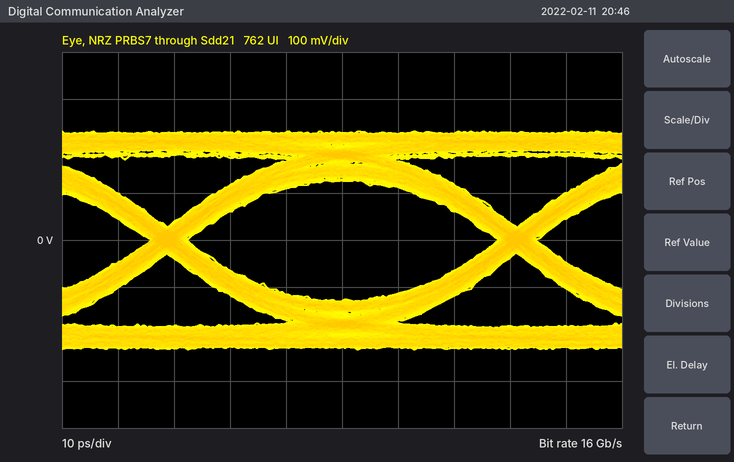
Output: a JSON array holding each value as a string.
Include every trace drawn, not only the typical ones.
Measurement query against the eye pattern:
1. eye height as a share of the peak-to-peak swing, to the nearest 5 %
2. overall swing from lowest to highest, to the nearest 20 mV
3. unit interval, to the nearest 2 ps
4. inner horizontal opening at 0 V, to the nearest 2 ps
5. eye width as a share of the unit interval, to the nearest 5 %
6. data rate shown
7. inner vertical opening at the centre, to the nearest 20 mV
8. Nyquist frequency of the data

["55 %", "460 mV", "62 ps", "56 ps", "90 %", "16 Gb/s", "260 mV", "8 GHz"]
